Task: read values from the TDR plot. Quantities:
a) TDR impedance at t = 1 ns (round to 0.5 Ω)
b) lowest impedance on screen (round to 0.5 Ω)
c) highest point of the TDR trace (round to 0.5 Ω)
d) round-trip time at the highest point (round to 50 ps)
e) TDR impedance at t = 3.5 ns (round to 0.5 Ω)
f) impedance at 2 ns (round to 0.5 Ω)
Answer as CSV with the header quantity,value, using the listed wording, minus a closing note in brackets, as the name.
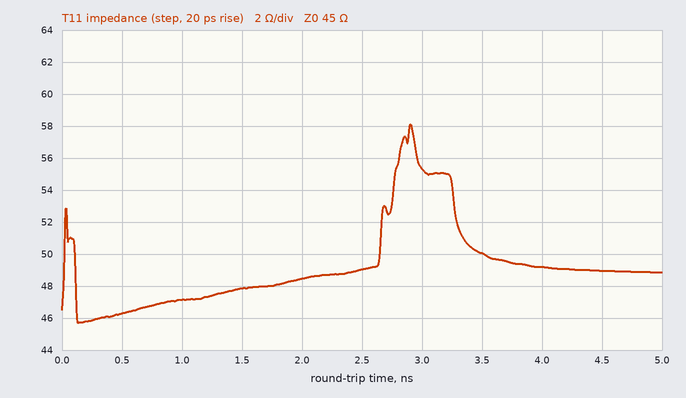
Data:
quantity,value
TDR impedance at t = 1 ns,47.0 Ω
lowest impedance on screen,45.5 Ω
highest point of the TDR trace,58.0 Ω
round-trip time at the highest point,2.90 ns
TDR impedance at t = 3.5 ns,50.0 Ω
impedance at 2 ns,48.5 Ω
